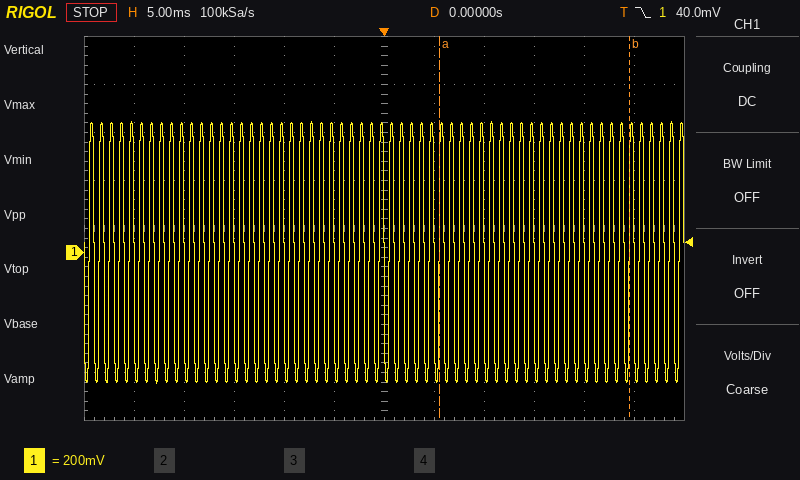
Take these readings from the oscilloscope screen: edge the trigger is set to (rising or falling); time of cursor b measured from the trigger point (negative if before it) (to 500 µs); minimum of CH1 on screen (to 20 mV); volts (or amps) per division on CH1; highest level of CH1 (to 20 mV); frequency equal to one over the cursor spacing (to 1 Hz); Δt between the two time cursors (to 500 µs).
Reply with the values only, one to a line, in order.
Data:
falling
+24.5 ms
-540 mV
200 mV
540 mV
53 Hz
19.0 ms
